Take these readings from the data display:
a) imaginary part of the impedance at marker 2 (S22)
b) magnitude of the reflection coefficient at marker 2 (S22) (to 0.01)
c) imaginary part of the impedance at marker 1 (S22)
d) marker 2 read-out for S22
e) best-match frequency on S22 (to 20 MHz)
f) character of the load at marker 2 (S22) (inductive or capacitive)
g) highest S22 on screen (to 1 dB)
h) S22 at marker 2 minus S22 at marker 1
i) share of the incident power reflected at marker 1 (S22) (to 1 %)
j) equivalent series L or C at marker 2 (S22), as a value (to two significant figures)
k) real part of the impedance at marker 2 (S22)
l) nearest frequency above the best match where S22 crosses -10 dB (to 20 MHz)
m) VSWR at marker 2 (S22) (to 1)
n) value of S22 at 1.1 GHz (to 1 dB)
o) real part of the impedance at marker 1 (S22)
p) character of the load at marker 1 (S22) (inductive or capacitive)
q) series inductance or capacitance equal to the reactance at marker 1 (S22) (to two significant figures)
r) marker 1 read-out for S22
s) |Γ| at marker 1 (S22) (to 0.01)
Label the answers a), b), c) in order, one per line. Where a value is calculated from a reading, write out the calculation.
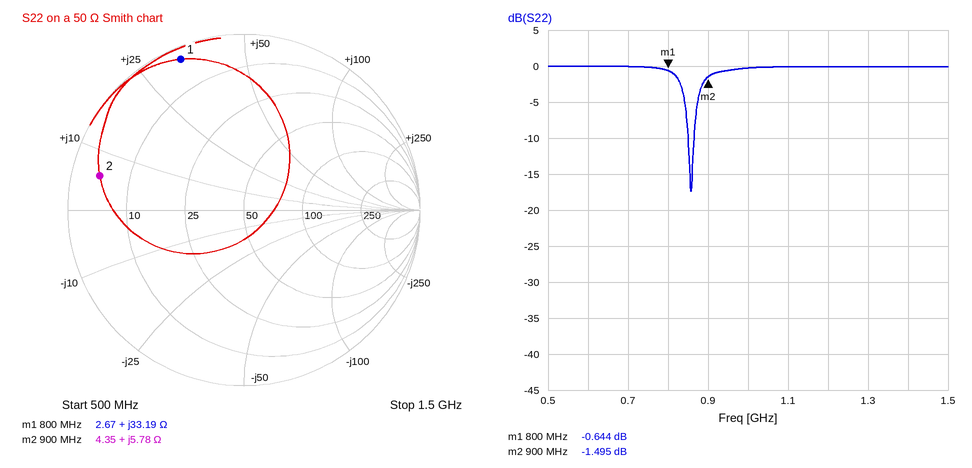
a) +5.78 Ω
b) 0.84
c) +33.19 Ω
d) -1.495 dB
e) 860 MHz
f) inductive
g) 0 dB
h) -1.495 − (-0.644) = -0.851 dB
i) 10^(-0.644/10) ≈ 86 %
j) L = 5.78 Ω/(2π × 900 MHz) ≈ 1.0 nH
k) 4.35 Ω
l) 860 MHz
m) (1 + 0.8419)/(1 − 0.8419) ≈ 12
n) 0 dB
o) 2.67 Ω
p) inductive
q) L = 33.19 Ω/(2π × 800 MHz) ≈ 6.6 nH
r) -0.644 dB
s) 0.93
